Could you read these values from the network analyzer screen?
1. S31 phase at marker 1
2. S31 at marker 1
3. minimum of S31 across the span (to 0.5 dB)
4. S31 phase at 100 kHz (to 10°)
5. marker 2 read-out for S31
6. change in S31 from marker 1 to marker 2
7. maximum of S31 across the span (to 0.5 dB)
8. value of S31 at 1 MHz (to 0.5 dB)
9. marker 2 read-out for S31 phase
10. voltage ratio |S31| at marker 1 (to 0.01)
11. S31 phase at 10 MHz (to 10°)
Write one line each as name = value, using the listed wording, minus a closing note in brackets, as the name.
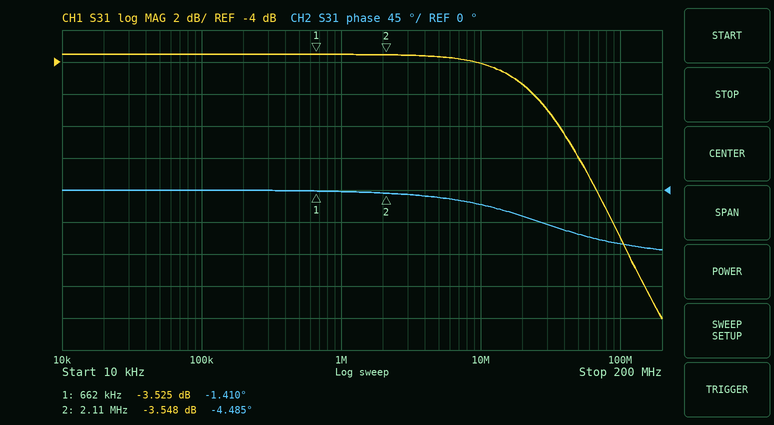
S31 phase at marker 1 = -1.410°
S31 at marker 1 = -3.525 dB
minimum of S31 across the span = -20.0 dB
S31 phase at 100 kHz = 0°
marker 2 read-out for S31 = -3.548 dB
change in S31 from marker 1 to marker 2 = -0.023 dB
maximum of S31 across the span = -3.5 dB
value of S31 at 1 MHz = -3.5 dB
marker 2 read-out for S31 phase = -4.485°
voltage ratio |S31| at marker 1 = 0.67
S31 phase at 10 MHz = -20°
